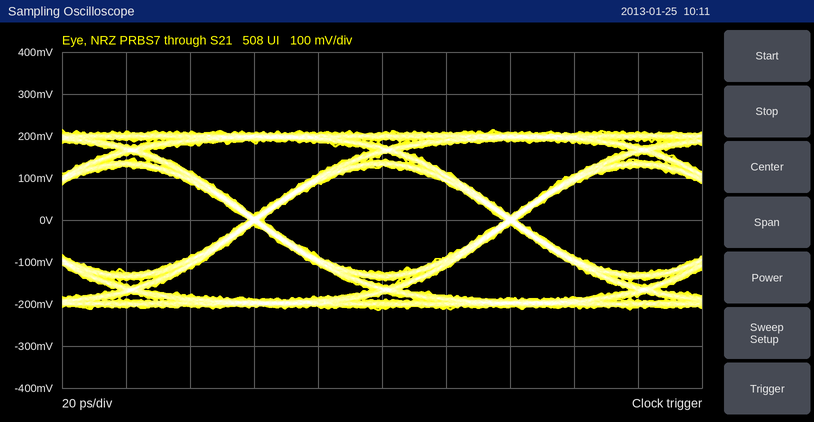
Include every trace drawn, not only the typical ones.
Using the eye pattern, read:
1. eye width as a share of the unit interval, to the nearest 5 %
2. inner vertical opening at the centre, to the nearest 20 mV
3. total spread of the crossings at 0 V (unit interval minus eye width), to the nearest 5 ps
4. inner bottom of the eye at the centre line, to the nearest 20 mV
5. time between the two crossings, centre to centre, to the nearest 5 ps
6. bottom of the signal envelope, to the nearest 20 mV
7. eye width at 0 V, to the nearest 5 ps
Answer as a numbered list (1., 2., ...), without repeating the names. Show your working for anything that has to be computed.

1. 75 ps / 80 ps ≈ 93.8 %, so 95 % to the nearest 5 %
2. 260 mV
3. 5 ps
4. -120 mV
5. 80 ps
6. -220 mV
7. 75 ps
